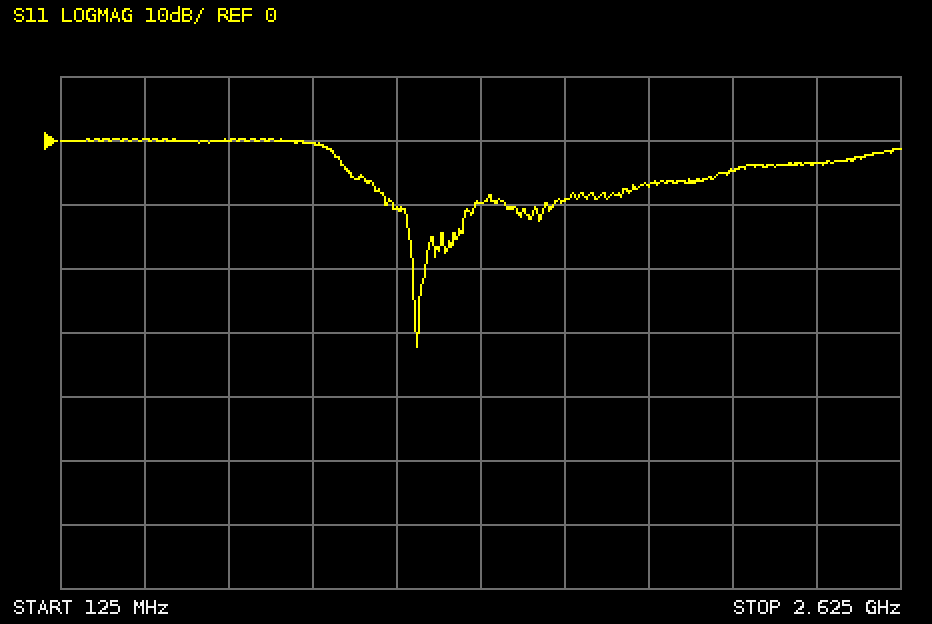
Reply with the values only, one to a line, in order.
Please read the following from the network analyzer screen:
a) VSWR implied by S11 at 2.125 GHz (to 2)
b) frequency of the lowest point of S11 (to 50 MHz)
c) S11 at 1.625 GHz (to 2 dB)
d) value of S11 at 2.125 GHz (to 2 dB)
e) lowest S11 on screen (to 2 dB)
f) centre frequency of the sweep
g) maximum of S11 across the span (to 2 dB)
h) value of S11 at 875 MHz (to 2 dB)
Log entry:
4
1.20 GHz
-10 dB
-4 dB
-32 dB
1.375 GHz
0 dB
0 dB
